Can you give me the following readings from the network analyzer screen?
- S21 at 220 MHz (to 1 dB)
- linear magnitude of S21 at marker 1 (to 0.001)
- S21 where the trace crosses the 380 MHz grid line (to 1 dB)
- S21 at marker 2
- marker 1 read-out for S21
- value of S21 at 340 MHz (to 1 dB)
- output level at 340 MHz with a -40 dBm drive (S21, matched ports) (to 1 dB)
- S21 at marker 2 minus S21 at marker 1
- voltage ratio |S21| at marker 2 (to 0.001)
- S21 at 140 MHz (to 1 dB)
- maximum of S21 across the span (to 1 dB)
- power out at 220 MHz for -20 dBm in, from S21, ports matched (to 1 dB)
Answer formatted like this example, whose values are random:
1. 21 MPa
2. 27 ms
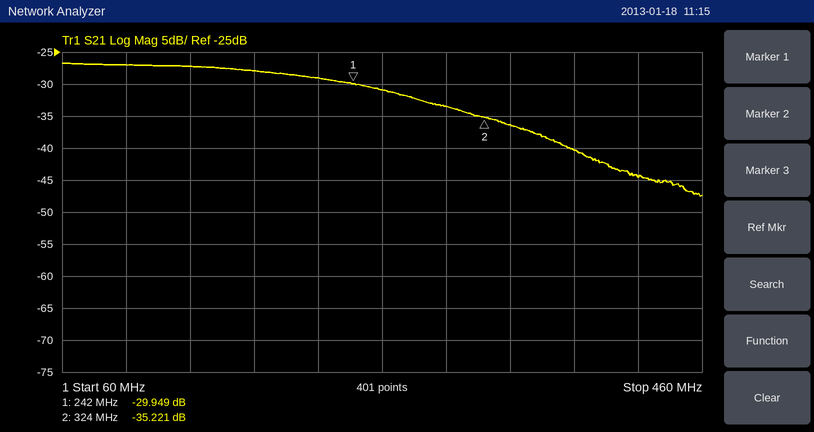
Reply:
1. -29 dB
2. 0.032
3. -40 dB
4. -35.221 dB
5. -29.949 dB
6. -36 dB
7. -76 dBm
8. -5.272 dB
9. 0.017
10. -27 dB
11. -27 dB
12. -49 dBm
